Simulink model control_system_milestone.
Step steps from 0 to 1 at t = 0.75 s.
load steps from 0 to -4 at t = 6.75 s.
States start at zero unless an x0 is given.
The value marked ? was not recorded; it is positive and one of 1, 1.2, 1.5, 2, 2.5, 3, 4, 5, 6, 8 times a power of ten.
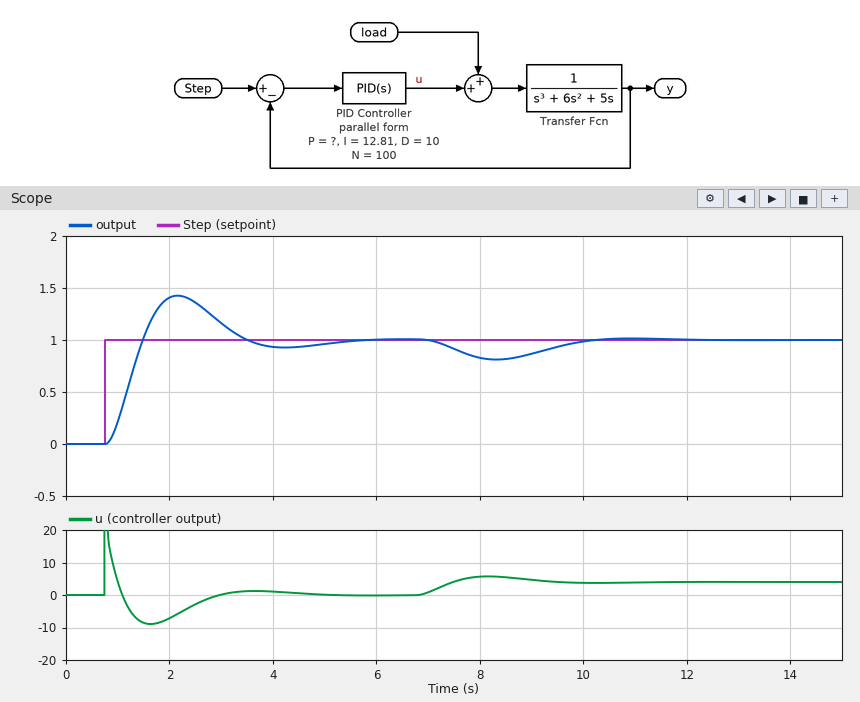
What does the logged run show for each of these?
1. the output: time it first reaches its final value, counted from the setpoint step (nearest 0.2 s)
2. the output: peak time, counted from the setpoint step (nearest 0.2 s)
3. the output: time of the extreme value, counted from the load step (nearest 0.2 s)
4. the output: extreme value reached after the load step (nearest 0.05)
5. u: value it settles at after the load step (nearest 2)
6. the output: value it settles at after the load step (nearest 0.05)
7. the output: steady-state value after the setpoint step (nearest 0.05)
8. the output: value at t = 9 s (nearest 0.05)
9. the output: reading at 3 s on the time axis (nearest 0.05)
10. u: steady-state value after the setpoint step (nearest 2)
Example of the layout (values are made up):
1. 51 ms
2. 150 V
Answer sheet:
1. 0.8 s
2. 1.4 s
3. 1.6 s
4. 0.80
5. 4
6. 1.00
7. 1.00
8. 0.85
9. 1.15
10. 0
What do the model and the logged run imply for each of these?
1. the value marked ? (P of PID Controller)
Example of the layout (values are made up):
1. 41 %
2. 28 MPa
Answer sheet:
1. 20
